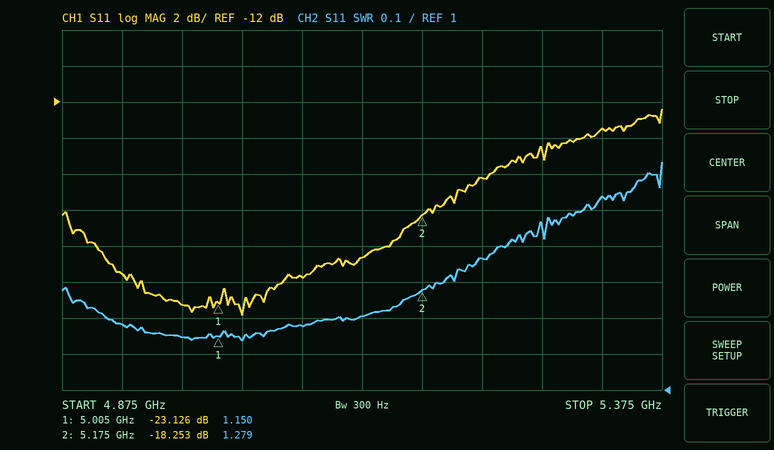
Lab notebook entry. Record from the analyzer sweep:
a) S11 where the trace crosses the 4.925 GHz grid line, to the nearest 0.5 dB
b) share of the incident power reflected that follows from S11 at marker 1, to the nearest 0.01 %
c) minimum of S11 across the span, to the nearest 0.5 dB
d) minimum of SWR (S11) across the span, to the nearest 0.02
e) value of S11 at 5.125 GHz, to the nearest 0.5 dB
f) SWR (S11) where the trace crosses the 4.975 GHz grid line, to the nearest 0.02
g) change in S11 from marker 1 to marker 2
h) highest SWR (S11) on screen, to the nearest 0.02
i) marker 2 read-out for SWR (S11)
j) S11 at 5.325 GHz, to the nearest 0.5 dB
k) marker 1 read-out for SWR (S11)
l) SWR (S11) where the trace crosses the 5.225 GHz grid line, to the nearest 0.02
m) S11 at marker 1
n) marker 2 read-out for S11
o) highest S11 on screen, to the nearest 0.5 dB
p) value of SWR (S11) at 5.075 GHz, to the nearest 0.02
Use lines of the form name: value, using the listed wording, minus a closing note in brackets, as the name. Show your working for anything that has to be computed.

S11 where the trace crosses the 4.925 GHz grid line, to the nearest 0.5 dB: -21.5 dB
share of the incident power reflected that follows from S11 at marker 1, to the nearest 0.01 %: 10^(-23.126/10) ≈ 0.49 %
minimum of S11 across the span, to the nearest 0.5 dB: -24.0 dB
minimum of SWR (S11) across the span, to the nearest 0.02: 1.14
value of S11 at 5.125 GHz, to the nearest 0.5 dB: -20.5 dB
SWR (S11) where the trace crosses the 4.975 GHz grid line, to the nearest 0.02: 1.14
change in S11 from marker 1 to marker 2: -18.253 − (-23.126) = 4.873 dB
highest SWR (S11) on screen, to the nearest 0.02: 1.64
marker 2 read-out for SWR: 1.279
S11 at 5.325 GHz, to the nearest 0.5 dB: -13.5 dB
marker 1 read-out for SWR: 1.150
SWR (S11) where the trace crosses the 5.225 GHz grid line, to the nearest 0.02: 1.36
S11 at marker 1: -23.126 dB
marker 2 read-out for S11: -18.253 dB
highest S11 on screen, to the nearest 0.5 dB: -12.5 dB
value of SWR (S11) at 5.075 GHz, to the nearest 0.02: 1.18
